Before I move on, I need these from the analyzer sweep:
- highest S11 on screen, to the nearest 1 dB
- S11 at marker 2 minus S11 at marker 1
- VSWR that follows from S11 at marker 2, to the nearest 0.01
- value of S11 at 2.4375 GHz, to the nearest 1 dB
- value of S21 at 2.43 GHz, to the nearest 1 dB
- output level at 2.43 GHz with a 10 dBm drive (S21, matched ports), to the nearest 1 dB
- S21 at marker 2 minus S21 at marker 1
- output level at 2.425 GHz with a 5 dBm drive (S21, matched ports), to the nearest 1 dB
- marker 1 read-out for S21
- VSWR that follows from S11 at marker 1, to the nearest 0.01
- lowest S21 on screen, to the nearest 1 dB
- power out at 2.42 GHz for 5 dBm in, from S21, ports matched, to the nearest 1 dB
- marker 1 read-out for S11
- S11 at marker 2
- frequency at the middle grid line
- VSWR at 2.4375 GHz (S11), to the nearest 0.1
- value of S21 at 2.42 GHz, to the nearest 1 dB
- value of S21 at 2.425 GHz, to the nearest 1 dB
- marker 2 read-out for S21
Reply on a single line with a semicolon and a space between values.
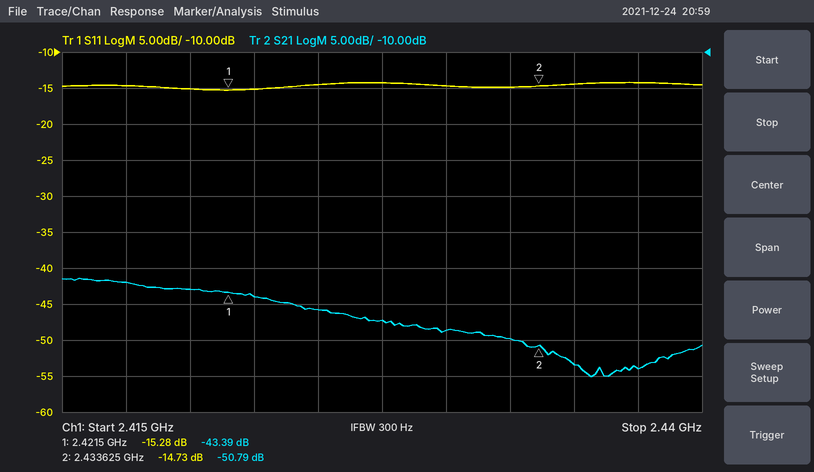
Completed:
-14 dB; 0.55 dB; 1.45; -14 dB; -49 dB; -39 dBm; -7.40 dB; -41 dBm; -43.39 dB; 1.42; -55 dB; -38 dBm; -15.28 dB; -14.73 dB; 2.4275 GHz; 1.5; -43 dB; -46 dB; -50.79 dB
